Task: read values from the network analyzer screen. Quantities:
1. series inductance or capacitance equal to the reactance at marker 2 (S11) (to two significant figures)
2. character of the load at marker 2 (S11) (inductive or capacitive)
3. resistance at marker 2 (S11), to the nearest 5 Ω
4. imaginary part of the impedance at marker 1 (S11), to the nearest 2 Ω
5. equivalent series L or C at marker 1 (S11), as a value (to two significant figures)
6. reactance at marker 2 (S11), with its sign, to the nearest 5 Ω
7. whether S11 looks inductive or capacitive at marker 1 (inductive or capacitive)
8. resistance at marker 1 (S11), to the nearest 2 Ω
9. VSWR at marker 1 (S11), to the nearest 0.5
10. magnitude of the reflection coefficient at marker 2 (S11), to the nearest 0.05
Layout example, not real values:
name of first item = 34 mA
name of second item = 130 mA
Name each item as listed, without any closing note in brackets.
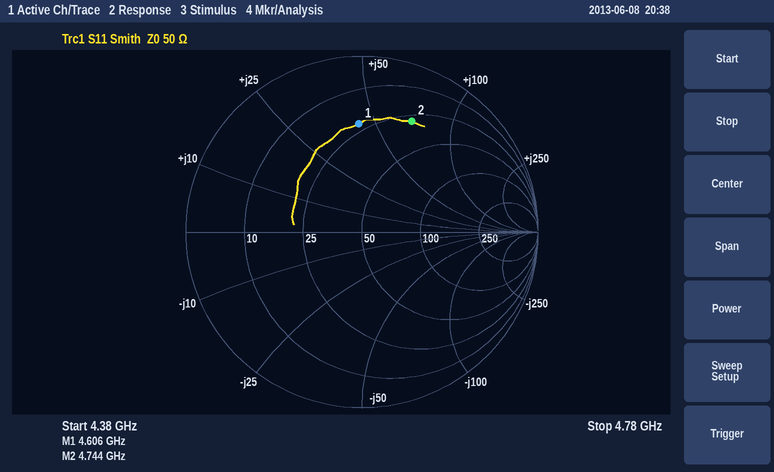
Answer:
series inductance or capacitance equal to the reactance at marker 2 (S11) = 2.3 nH
character of the load at marker 2 (S11) = inductive
resistance at marker 2 (S11), to the nearest 5 Ω = 30 Ω
imaginary part of the impedance at marker 1 (S11), to the nearest 2 Ω = +44 Ω
equivalent series L or C at marker 1 (S11), as a value = 1.5 nH
reactance at marker 2 (S11), with its sign, to the nearest 5 Ω = +70 Ω
whether S11 looks inductive or capacitive at marker 1 = inductive
resistance at marker 1 (S11), to the nearest 2 Ω = 22 Ω
VSWR at marker 1 (S11), to the nearest 0.5 = 4.0
magnitude of the reflection coefficient at marker 2 (S11), to the nearest 0.05 = 0.70
